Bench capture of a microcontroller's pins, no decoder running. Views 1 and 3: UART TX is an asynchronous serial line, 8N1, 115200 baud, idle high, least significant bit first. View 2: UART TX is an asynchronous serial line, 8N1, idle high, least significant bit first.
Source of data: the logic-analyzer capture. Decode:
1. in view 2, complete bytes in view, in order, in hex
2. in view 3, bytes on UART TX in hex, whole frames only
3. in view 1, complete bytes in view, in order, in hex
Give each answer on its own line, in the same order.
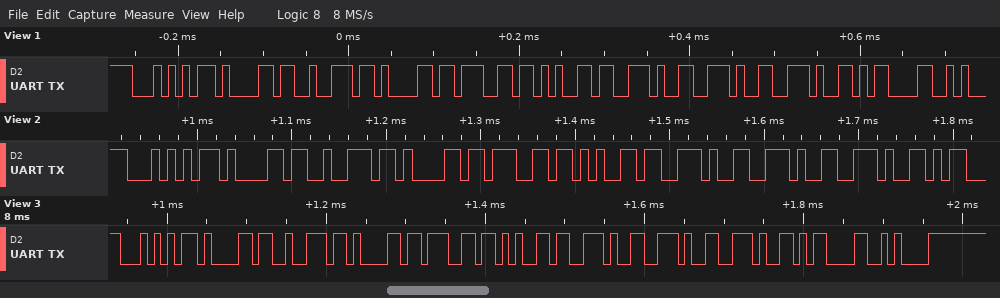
54 61 72 61 67 65 2E 2E 2E
54 61 72 61 67 65 2E 2E 2E 0D 0A
54 61 72 61 67 65 2E 2E 2E 0D
